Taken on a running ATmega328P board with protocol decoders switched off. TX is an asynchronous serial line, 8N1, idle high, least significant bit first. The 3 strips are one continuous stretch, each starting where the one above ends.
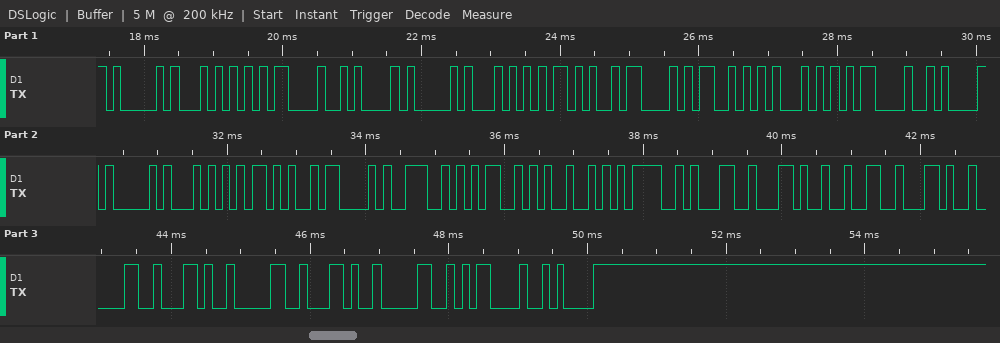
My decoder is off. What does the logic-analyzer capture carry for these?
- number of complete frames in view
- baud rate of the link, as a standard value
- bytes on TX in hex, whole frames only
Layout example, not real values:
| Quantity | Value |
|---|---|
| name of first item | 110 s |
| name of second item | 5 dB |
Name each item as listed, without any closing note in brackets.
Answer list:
| Quantity | Value |
|---|---|
| number of complete frames in view | 31 |
| baud rate of the link, as a standard value | 9600 baud |
| bytes on TX in hex, whole frames only | 0x41 0x54 0x0D 0x0A 0x41 0x54 0x2B 0x43 0x53 0x51 0x0D 0x0A 0x41 0x54 0x2B 0x43 0x4E 0x4D 0x49 0x3D 0x31 0x2C 0x32 0x2C 0x30 0x2C 0x30 0x2C 0x30 0x0D 0x0A |
